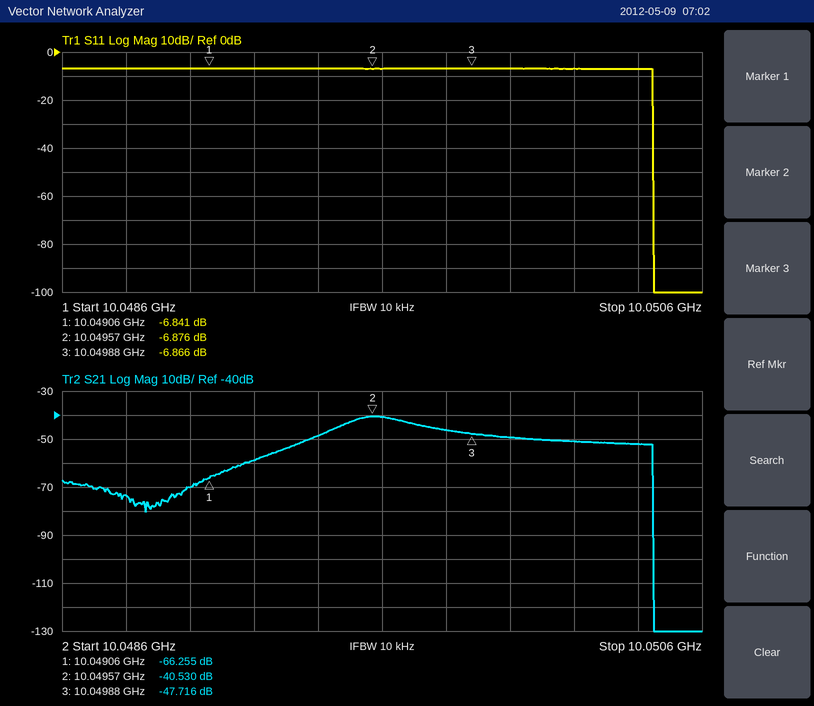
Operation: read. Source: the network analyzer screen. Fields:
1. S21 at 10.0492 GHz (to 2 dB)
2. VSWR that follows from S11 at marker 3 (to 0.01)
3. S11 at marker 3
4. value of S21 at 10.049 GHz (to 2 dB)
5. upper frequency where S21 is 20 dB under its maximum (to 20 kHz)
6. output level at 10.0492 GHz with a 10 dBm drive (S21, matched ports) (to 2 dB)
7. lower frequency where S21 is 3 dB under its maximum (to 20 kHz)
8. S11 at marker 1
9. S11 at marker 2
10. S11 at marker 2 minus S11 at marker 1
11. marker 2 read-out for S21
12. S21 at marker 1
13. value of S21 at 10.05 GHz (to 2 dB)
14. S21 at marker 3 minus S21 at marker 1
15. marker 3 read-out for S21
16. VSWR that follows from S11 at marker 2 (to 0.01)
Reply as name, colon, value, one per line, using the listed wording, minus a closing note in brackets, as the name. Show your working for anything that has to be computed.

S21 at 10.0492 GHz: -58 dB
VSWR that follows from S11 at marker 3: (1 + 0.4536)/(1 − 0.4536) ≈ 2.66
S11 at marker 3: -6.866 dB
value of S21 at 10.049 GHz: -70 dB
upper frequency where S21 is 20 dB under its maximum: 10.05044 GHz
output level at 10.0492 GHz with a 10 dBm drive (S21, matched ports): 10 dBm + (-58 dB) = -48 dBm
lower frequency where S21 is 3 dB under its maximum: 10.04948 GHz
S11 at marker 1: -6.841 dB
S11 at marker 2: -6.876 dB
S11 at marker 2 minus S11 at marker 1: -6.876 − (-6.841) = -0.035 dB
marker 2 read-out for S21: -40.530 dB
S21 at marker 1: -66.255 dB
value of S21 at 10.05 GHz: -50 dB
S21 at marker 3 minus S21 at marker 1: -47.716 − (-66.255) = 18.539 dB
marker 3 read-out for S21: -47.716 dB
VSWR that follows from S11 at marker 2: (1 + 0.4531)/(1 − 0.4531) ≈ 2.66
